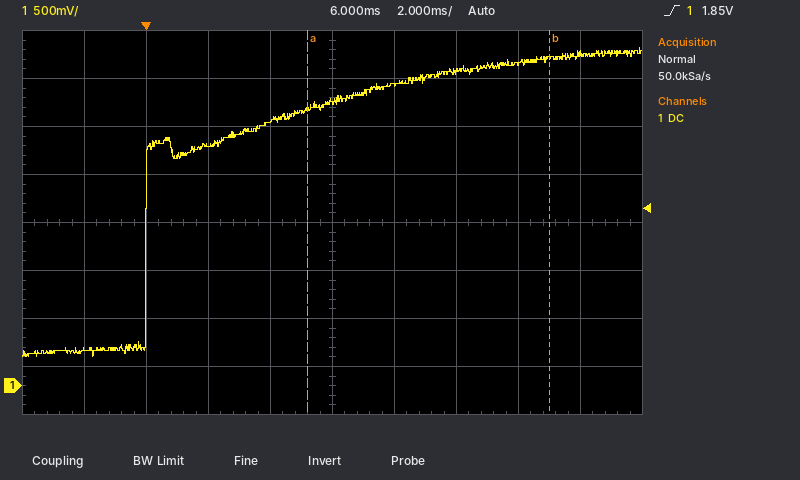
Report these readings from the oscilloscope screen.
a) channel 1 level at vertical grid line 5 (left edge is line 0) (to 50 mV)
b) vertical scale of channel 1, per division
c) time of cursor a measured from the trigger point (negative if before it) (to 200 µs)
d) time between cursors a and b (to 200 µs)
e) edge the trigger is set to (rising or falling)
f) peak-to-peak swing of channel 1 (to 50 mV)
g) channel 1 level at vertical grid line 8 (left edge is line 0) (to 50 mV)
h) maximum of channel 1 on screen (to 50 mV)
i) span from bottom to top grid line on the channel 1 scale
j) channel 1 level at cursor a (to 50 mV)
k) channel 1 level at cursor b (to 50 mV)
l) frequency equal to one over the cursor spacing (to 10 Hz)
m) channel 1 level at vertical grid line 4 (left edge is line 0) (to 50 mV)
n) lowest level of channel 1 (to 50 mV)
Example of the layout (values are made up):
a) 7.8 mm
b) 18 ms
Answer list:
a) 2.95 V
b) 500 mV
c) +5.2 ms
d) 7.8 ms
e) rising
f) 3.20 V
g) 3.35 V
h) 3.50 V
i) 4 V
j) 2.90 V
k) 3.40 V
l) 130 Hz
m) 2.75 V
n) 300 mV
